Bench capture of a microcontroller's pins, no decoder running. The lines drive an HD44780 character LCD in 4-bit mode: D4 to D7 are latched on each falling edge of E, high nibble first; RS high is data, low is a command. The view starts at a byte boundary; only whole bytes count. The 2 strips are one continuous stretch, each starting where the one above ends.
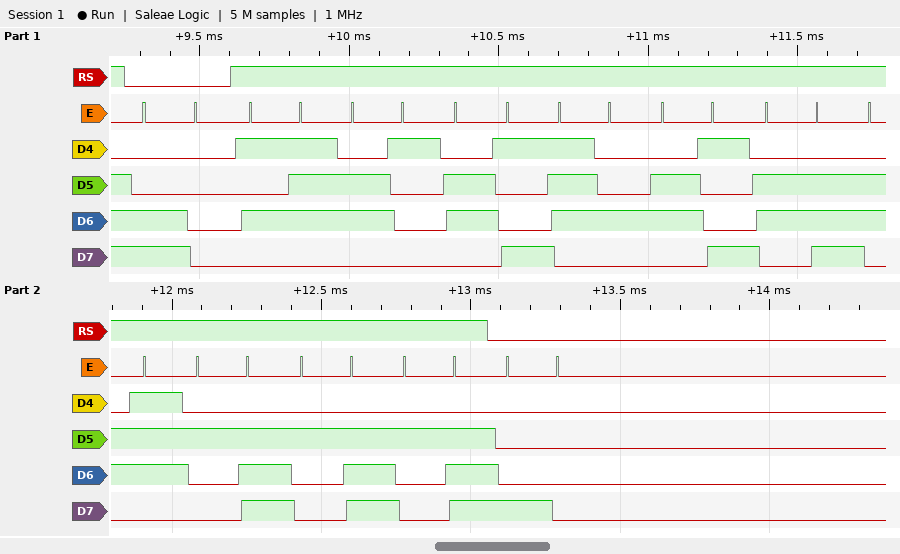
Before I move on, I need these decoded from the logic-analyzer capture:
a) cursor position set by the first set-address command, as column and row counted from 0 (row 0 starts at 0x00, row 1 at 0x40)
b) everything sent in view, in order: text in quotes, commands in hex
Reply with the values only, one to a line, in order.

column 0, row 1
0xC0 "Waiting..." 0x80
